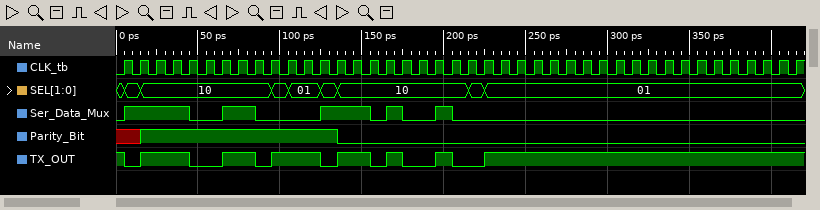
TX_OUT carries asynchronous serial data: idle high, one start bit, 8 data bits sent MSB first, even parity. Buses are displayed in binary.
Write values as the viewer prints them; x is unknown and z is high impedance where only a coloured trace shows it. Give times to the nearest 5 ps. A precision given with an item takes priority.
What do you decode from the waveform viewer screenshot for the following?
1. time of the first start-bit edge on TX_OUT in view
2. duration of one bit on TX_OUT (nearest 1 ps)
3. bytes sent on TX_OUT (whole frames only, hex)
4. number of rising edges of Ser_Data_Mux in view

5 ps
10 ps
E6, D2
5
